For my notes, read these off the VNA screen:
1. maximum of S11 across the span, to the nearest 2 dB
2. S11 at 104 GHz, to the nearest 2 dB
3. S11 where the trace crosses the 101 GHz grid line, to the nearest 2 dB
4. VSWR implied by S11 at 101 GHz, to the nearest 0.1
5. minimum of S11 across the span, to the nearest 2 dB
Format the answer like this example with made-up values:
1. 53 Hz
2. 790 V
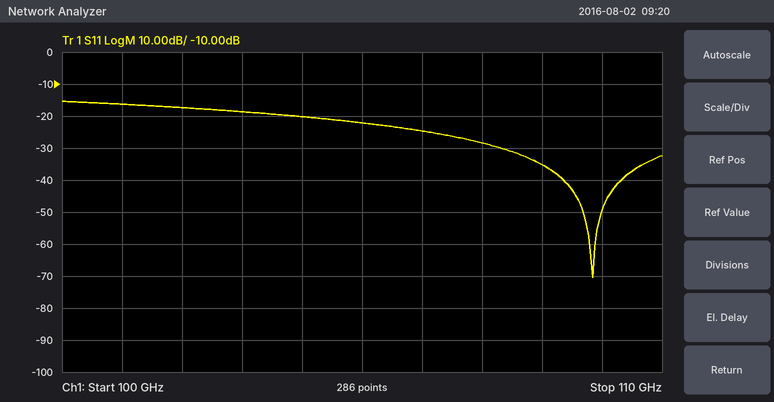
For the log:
1. -16 dB
2. -20 dB
3. -16 dB
4. 1.4
5. -70 dB
